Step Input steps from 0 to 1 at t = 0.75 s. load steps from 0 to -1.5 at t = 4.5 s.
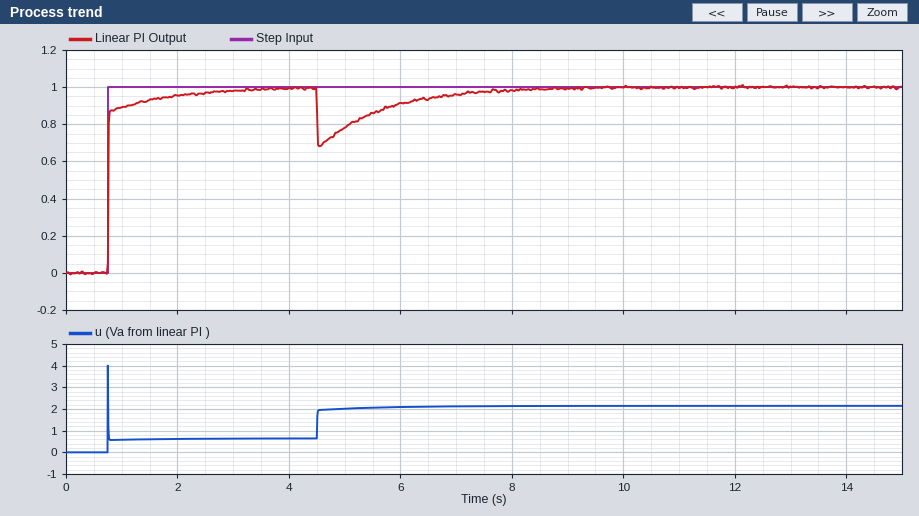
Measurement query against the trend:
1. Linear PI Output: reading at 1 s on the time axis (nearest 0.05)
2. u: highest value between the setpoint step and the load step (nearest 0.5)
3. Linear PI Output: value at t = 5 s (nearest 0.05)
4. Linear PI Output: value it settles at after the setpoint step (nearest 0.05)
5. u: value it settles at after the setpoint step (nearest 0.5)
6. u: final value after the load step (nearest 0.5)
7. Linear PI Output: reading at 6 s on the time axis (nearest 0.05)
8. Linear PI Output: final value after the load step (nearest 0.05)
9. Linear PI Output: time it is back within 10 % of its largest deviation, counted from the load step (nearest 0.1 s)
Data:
0.90
4.0
0.80
1.00
0.5
2.0
0.90
1.00
2.7 s
